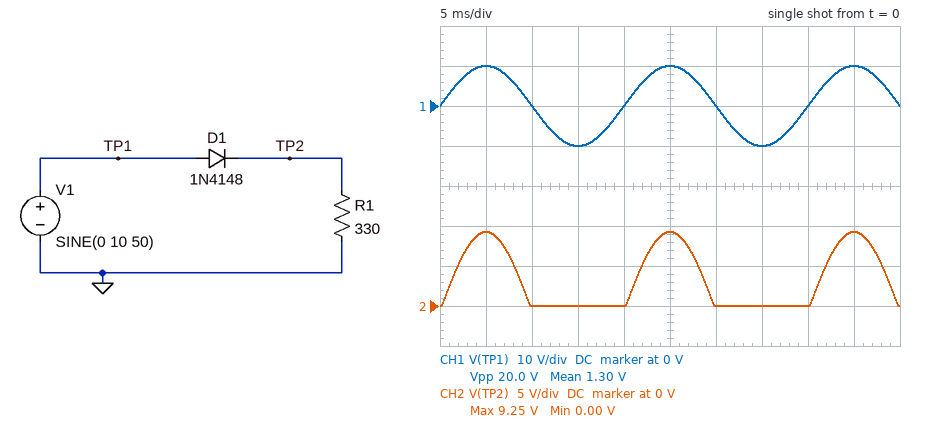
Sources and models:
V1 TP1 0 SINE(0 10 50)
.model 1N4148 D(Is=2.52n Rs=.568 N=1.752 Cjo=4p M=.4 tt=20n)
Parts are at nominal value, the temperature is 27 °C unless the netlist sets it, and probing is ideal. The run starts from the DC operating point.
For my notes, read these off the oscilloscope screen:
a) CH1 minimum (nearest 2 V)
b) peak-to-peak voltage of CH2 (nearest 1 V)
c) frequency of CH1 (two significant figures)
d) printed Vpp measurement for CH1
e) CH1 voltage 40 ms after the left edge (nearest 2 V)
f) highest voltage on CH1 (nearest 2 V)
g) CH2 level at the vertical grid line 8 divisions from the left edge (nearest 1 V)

-10 V
9 V
50 Hz
20.0 V
0 V
10 V
0 V
